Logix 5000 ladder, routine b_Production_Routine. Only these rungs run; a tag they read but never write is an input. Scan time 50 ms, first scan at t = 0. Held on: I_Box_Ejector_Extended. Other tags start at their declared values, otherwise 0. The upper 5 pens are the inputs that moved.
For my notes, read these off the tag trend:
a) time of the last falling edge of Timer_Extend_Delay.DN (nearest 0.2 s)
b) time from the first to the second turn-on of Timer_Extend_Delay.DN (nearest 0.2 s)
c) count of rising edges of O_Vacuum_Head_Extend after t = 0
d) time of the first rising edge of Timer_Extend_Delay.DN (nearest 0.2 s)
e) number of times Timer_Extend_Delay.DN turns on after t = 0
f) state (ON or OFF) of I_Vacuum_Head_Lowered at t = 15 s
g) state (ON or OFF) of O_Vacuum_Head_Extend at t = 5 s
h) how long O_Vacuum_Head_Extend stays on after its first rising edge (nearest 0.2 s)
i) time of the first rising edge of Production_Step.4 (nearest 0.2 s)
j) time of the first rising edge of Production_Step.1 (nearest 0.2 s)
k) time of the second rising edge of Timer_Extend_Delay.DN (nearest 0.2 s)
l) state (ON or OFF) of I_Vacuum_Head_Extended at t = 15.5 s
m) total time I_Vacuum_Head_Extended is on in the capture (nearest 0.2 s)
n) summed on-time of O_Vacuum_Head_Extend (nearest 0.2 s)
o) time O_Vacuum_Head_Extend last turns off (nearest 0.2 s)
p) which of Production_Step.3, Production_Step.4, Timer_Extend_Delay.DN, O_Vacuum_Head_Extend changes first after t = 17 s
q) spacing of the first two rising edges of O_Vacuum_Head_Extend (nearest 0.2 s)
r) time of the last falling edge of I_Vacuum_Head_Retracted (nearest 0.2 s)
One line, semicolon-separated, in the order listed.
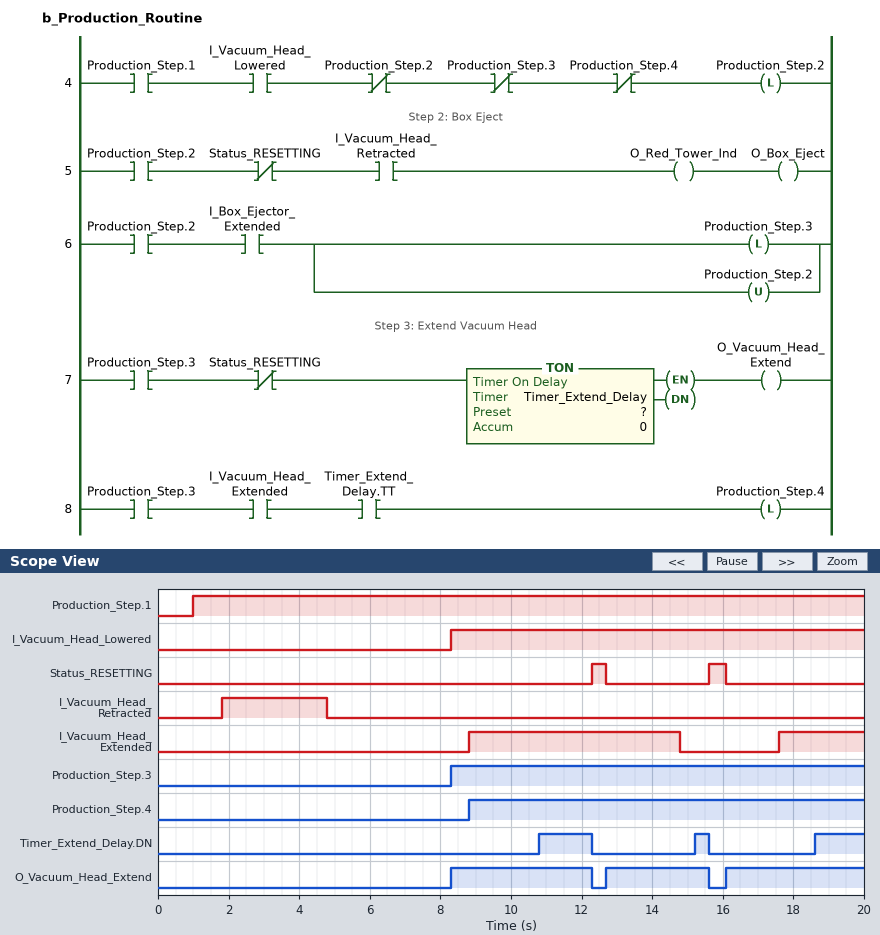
15.6 s; 4.4 s; 3; 10.8 s; 3; ON; OFF; 4.0 s; 8.8 s; 1.0 s; 15.2 s; OFF; 8.4 s; 10.8 s; 15.6 s; Timer_Extend_Delay.DN; 4.4 s; 4.8 s
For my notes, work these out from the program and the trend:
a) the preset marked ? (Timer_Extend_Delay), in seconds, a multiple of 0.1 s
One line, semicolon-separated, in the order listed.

2.5 s
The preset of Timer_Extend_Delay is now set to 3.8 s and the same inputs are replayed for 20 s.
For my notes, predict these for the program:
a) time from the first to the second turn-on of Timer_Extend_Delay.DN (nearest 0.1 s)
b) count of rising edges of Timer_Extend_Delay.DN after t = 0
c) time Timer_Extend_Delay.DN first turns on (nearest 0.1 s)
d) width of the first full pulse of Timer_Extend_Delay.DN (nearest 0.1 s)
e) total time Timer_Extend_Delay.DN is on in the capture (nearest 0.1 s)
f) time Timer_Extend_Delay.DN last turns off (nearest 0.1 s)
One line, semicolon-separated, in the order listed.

7.8 s; 2; 12.1 s; 0.2 s; 0.3 s; 12.3 s
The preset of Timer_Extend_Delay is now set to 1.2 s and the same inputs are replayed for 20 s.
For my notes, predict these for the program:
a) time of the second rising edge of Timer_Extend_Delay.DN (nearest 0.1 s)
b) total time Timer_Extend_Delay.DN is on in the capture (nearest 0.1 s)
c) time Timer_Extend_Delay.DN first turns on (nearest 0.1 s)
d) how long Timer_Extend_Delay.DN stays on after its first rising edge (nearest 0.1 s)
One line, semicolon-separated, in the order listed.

13.9 s; 7.2 s; 9.5 s; 2.8 s
